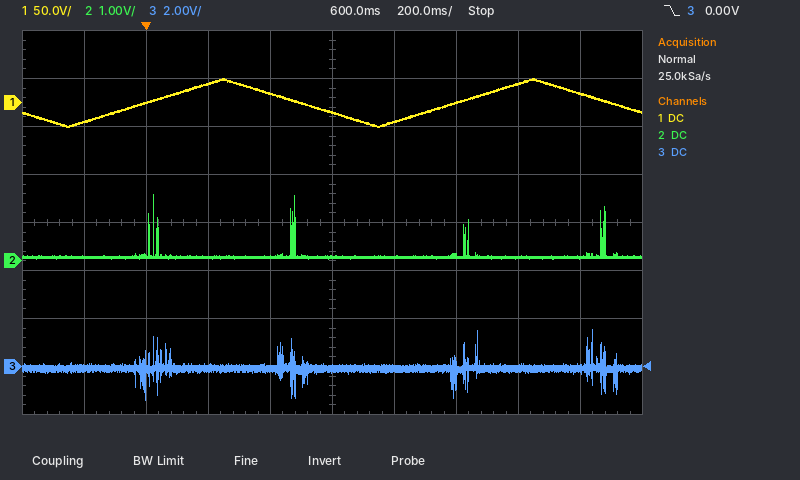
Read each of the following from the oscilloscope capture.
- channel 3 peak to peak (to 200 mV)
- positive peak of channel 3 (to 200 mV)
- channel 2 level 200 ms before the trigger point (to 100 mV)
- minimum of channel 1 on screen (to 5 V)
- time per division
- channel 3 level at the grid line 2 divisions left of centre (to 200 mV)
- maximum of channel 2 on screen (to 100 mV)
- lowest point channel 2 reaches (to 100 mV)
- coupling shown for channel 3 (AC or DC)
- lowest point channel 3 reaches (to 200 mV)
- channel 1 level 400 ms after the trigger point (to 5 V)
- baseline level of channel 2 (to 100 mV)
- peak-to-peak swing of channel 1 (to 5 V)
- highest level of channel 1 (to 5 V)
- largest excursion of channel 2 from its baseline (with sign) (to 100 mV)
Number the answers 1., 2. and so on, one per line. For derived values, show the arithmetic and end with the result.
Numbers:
1. 1.6 V − (-1.4 V) = 3.0 V
2. 1.6 V
3. 100 mV
4. -25 V
5. 200 ms
6. 0.0 V
7. 1.4 V
8. 0.0 V
9. DC
10. -1.4 V
11. 10 V
12. 100 mV
13. 25 V − (-25 V) = 50 V
14. 25 V
15. 1.4 V − (100 mV) = +1.3 V
